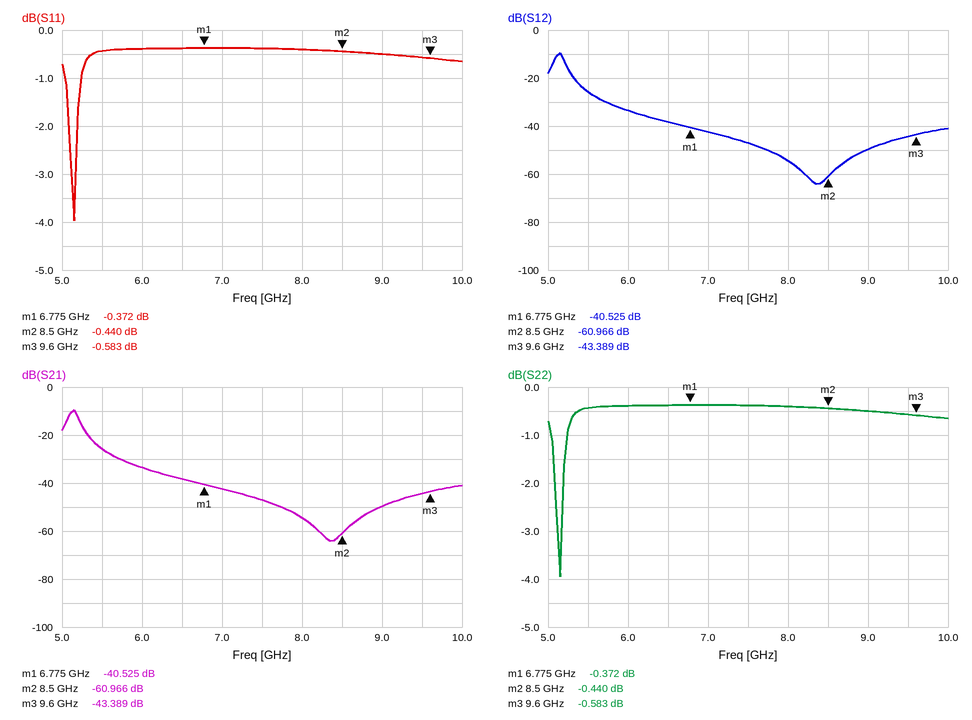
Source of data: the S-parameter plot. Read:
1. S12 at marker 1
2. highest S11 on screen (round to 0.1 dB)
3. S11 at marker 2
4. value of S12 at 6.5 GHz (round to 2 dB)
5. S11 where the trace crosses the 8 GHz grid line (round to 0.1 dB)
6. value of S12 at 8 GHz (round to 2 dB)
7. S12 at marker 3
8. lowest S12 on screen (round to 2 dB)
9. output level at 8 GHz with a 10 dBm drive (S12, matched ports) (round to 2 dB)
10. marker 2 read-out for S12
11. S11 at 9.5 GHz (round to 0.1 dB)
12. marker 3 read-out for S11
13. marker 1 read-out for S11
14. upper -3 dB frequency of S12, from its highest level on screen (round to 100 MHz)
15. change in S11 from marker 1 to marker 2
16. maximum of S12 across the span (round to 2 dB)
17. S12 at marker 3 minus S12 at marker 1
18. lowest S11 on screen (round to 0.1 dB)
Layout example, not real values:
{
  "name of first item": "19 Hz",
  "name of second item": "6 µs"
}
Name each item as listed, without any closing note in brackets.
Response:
{
  "S12 at marker 1": "-40.525 dB",
  "highest S11 on screen": "-0.4 dB",
  "S11 at marker 2": "-0.440 dB",
  "value of S12 at 6.5 GHz": "-38 dB",
  "S11 where the trace crosses the 8 GHz grid line": "-0.4 dB",
  "value of S12 at 8 GHz": "-54 dB",
  "S12 at marker 3": "-43.389 dB",
  "lowest S12 on screen": "-64 dB",
  "output level at 8 GHz with a 10 dBm drive (S12, matched ports)": "-44 dBm",
  "marker 2 read-out for S12": "-60.966 dB",
  "S11 at 9.5 GHz": "-0.6 dB",
  "marker 3 read-out for S11": "-0.583 dB",
  "marker 1 read-out for S11": "-0.372 dB",
  "upper -3 dB frequency of S12, from its highest level on screen": "5.2 GHz",
  "change in S11 from marker 1 to marker 2": "-0.068 dB",
  "maximum of S12 across the span": "-10 dB",
  "S12 at marker 3 minus S12 at marker 1": "-2.864 dB",
  "lowest S11 on screen": "-4.0 dB"
}
